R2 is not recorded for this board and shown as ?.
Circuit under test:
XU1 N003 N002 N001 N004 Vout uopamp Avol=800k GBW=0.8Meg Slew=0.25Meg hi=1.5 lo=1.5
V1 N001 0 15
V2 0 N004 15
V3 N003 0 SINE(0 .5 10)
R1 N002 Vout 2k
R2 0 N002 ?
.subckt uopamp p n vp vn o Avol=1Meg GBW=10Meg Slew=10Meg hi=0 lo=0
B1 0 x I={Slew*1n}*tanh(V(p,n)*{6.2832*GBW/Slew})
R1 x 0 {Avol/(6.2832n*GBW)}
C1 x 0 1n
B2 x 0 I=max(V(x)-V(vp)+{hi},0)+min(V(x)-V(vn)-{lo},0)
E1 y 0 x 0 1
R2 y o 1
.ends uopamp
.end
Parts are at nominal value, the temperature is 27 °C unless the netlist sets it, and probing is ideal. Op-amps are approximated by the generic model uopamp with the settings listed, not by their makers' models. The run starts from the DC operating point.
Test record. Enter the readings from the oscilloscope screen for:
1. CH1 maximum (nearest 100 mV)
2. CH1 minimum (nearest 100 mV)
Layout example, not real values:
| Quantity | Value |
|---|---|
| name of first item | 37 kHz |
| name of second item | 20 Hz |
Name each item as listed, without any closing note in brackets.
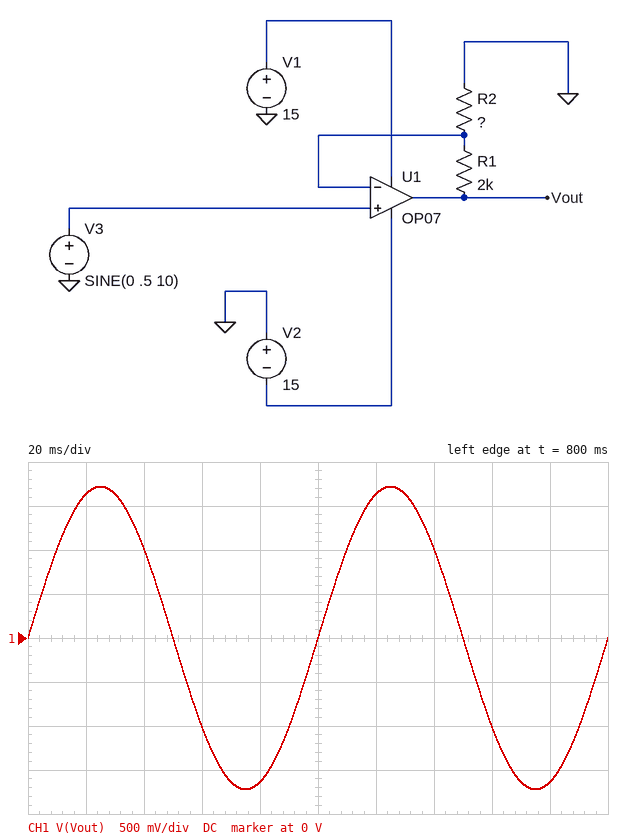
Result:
| Quantity | Value |
|---|---|
| CH1 maximum | 1.7 V |
| CH1 minimum | -1.7 V |
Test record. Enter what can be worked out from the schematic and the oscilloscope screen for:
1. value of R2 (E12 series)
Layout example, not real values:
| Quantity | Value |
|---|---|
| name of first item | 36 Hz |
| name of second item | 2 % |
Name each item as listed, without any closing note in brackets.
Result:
| Quantity | Value |
|---|---|
| value of R2 | 820 Ω |
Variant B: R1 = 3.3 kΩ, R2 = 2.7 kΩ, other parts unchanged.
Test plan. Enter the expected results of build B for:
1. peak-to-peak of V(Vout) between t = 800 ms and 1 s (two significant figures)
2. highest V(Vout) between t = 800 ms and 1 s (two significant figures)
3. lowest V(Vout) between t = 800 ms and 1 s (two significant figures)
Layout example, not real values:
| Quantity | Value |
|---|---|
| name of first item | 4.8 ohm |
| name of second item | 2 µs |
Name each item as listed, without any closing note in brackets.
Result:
| Quantity | Value |
|---|---|
| peak-to-peak of V(Vout) between t = 800 ms and 1 s | 2.2 V |
| highest V(Vout) between t = 800 ms and 1 s | 1.1 V |
| lowest V(Vout) between t = 800 ms and 1 s | -1.1 V |
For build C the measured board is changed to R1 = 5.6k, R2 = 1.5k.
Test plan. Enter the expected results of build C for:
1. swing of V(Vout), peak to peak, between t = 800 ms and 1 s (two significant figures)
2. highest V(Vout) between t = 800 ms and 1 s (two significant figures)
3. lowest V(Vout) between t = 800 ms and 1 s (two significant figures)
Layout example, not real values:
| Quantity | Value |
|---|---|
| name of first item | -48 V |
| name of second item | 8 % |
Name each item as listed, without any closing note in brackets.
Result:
| Quantity | Value |
|---|---|
| swing of V(Vout), peak to peak, between t = 800 ms and 1 s | 4.7 V |
| highest V(Vout) between t = 800 ms and 1 s | 2.4 V |
| lowest V(Vout) between t = 800 ms and 1 s | -2.4 V |
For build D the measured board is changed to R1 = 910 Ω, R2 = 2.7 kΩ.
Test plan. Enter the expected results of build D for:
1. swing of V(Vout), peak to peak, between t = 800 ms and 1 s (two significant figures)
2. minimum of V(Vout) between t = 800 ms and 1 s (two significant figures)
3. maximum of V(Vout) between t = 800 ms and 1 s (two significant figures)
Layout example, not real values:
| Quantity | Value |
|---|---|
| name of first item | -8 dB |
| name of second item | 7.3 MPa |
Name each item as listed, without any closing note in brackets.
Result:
| Quantity | Value |
|---|---|
| swing of V(Vout), peak to peak, between t = 800 ms and 1 s | 1.3 V |
| minimum of V(Vout) between t = 800 ms and 1 s | -670 mV |
| maximum of V(Vout) between t = 800 ms and 1 s | 670 mV |
